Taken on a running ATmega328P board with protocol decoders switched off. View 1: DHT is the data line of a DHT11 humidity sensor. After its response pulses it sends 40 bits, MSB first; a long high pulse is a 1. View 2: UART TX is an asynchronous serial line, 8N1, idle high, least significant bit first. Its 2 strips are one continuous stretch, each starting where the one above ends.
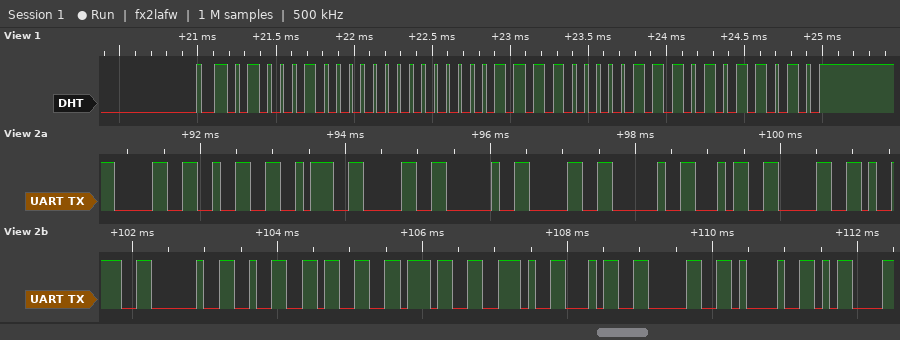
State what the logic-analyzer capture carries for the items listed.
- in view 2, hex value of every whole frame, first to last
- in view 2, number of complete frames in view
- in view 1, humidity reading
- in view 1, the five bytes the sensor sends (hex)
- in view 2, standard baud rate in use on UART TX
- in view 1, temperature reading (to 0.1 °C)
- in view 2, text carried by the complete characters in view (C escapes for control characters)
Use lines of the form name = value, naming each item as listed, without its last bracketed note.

in view 2, hex value of every whole frame, first to last = 0x30 0x32 0x3A 0x30 0x20 0x30 0x20 0x34 0x30 0x39 0x20 0x32 0x33 0x37 0x2E 0x34 0x30 0x21 0x0D
in view 2, number of complete frames in view = 19
in view 1, humidity reading = 68 %
in view 1, the five bytes the sensor sends = 44 00 0F 07 5A
in view 2, standard baud rate in use on UART TX = 9600 baud
in view 1, temperature reading = 15.7 °C
in view 2, text carried by the complete characters in view = "02:0 0 409 237.40!\r"
